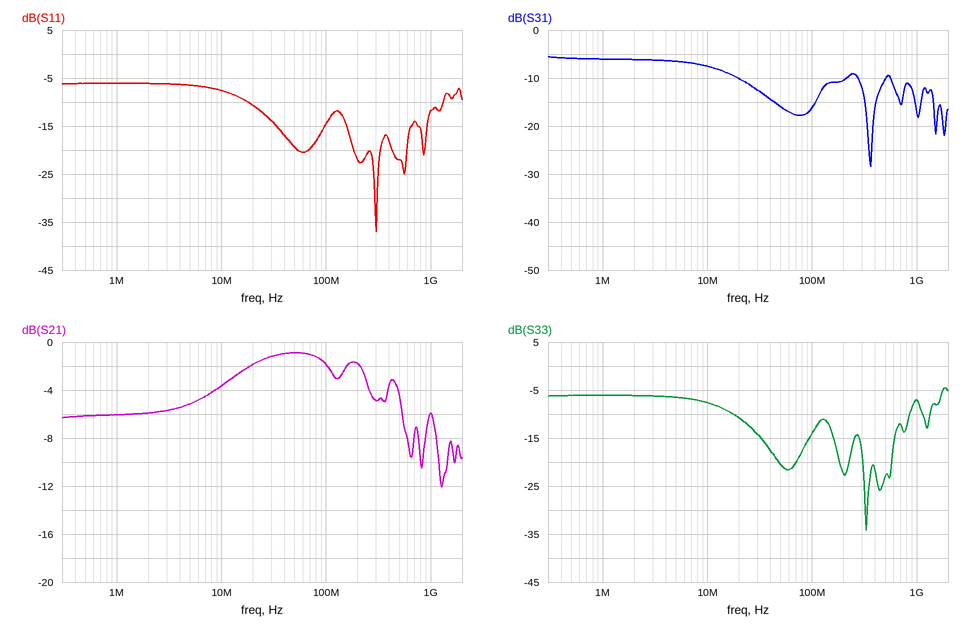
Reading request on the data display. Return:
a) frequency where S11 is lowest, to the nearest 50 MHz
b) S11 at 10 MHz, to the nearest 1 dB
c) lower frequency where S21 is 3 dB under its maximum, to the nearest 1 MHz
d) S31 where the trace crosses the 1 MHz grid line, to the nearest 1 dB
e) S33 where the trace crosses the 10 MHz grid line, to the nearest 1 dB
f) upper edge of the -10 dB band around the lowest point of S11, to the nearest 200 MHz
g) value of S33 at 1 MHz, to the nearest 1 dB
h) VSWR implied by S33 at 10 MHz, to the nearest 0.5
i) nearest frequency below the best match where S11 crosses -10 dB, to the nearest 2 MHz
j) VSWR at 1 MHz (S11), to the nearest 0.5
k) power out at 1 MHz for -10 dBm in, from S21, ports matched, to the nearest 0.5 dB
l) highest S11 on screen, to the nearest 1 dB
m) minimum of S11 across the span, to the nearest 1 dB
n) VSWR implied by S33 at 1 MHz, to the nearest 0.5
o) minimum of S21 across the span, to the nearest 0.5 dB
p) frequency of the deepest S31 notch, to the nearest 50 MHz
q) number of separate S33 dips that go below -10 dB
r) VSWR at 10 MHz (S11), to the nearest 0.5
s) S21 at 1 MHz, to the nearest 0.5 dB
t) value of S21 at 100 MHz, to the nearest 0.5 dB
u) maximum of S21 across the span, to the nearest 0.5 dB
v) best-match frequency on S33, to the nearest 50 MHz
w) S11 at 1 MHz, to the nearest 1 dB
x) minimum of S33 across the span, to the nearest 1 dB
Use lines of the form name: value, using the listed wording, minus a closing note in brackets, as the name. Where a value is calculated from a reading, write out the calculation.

frequency where S11 is lowest, to the nearest 50 MHz: 300 MHz
S11 at 10 MHz, to the nearest 1 dB: -8 dB
lower frequency where S21 is 3 dB under its maximum, to the nearest 1 MHz: 9 MHz
S31 where the trace crosses the 1 MHz grid line, to the nearest 1 dB: -6 dB
S33 where the trace crosses the 10 MHz grid line, to the nearest 1 dB: -8 dB
upper edge of the -10 dB band around the lowest point of S11, to the nearest 200 MHz: 1.4 GHz
value of S33 at 1 MHz, to the nearest 1 dB: -6 dB
VSWR implied by S33 at 10 MHz, to the nearest 0.5: |Γ| = 10^(-8/20) = 0.3981; VSWR = (1 + 0.3981)/(1 − 0.3981) ≈ 2.32, so 2.5 to the nearest 0.5
nearest frequency below the best match where S11 crosses -10 dB, to the nearest 2 MHz: 18 MHz
VSWR at 1 MHz (S11), to the nearest 0.5: |Γ| = 10^(-6/20) = 0.5012; VSWR = (1 + 0.5012)/(1 − 0.5012) ≈ 3.0
power out at 1 MHz for -10 dBm in, from S21, ports matched, to the nearest 0.5 dB: -10 dBm + (-6.0 dB) = -16.0 dBm
highest S11 on screen, to the nearest 1 dB: -6 dB
minimum of S11 across the span, to the nearest 1 dB: -37 dB
VSWR implied by S33 at 1 MHz, to the nearest 0.5: |Γ| = 10^(-6/20) = 0.5012; VSWR = (1 + 0.5012)/(1 − 0.5012) ≈ 3.0
minimum of S21 across the span, to the nearest 0.5 dB: -12.0 dB
frequency of the deepest S31 notch, to the nearest 50 MHz: 350 MHz
number of separate S33 dips that go below -10 dB: 5
VSWR at 10 MHz (S11), to the nearest 0.5: |Γ| = 10^(-8/20) = 0.3981; VSWR = (1 + 0.3981)/(1 − 0.3981) ≈ 2.32, so 2.5 to the nearest 0.5
S21 at 1 MHz, to the nearest 0.5 dB: -6.0 dB
value of S21 at 100 MHz, to the nearest 0.5 dB: -2.0 dB
maximum of S21 across the span, to the nearest 0.5 dB: -1.0 dB
best-match frequency on S33, to the nearest 50 MHz: 350 MHz
S11 at 1 MHz, to the nearest 1 dB: -6 dB
minimum of S33 across the span, to the nearest 1 dB: -34 dB
